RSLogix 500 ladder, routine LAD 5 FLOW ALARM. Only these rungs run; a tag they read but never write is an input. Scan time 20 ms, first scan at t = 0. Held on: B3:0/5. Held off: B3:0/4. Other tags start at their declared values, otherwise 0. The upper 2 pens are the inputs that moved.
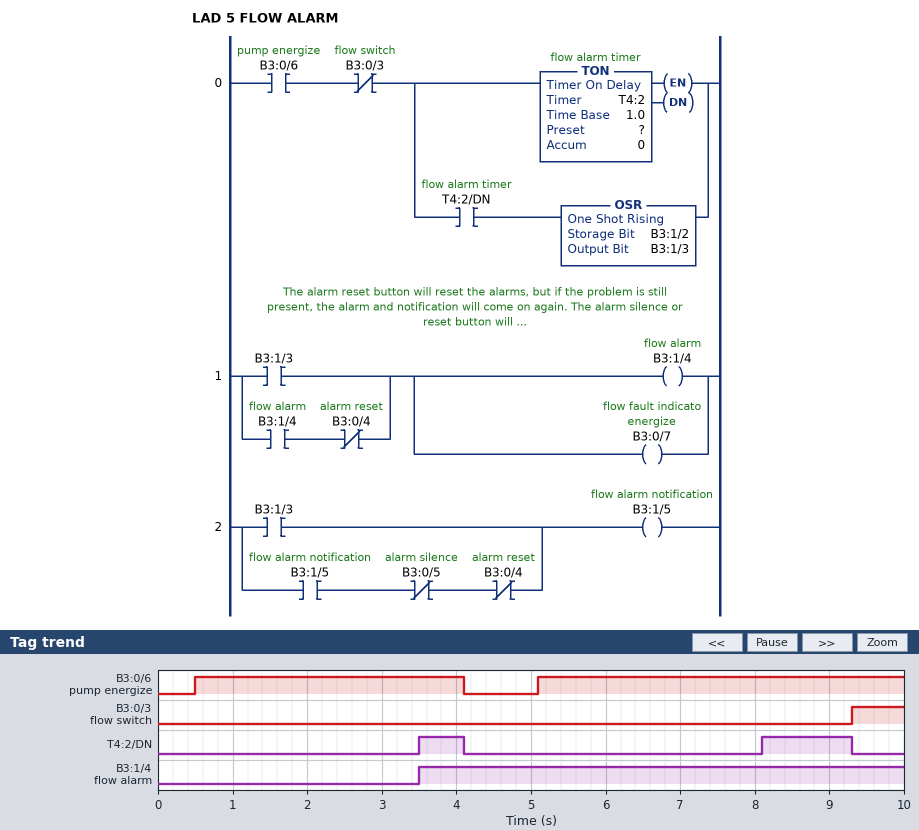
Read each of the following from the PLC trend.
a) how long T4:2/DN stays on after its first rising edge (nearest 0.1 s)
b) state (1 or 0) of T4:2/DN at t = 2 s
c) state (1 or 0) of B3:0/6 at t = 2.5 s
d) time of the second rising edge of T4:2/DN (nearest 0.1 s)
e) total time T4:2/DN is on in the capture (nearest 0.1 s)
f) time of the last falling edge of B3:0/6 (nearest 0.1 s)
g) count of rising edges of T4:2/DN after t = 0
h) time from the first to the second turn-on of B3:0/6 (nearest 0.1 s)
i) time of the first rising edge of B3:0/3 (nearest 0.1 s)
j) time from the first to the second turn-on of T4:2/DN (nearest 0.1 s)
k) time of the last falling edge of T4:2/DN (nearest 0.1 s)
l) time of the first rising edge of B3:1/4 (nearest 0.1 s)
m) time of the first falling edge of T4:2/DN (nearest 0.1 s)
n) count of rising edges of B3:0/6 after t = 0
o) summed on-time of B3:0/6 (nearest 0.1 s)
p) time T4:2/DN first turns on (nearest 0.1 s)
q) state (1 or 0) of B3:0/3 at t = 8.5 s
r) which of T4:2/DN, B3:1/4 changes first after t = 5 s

0.6 s
0
1
8.1 s
1.8 s
4.1 s
2
4.6 s
9.3 s
4.6 s
9.3 s
3.5 s
4.1 s
2
8.5 s
3.5 s
0
T4:2/DN
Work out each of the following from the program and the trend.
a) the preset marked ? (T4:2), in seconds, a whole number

3 s
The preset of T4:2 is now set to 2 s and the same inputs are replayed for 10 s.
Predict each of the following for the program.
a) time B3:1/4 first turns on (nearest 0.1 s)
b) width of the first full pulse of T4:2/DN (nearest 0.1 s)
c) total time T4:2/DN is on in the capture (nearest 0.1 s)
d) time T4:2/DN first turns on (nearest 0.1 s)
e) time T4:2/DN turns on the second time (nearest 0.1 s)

2.5 s
1.6 s
3.8 s
2.5 s
7.1 s
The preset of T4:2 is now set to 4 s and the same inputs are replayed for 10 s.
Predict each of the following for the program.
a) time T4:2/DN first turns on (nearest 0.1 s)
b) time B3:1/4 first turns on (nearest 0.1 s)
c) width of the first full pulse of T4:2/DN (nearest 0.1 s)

9.1 s
9.1 s
0.2 s
